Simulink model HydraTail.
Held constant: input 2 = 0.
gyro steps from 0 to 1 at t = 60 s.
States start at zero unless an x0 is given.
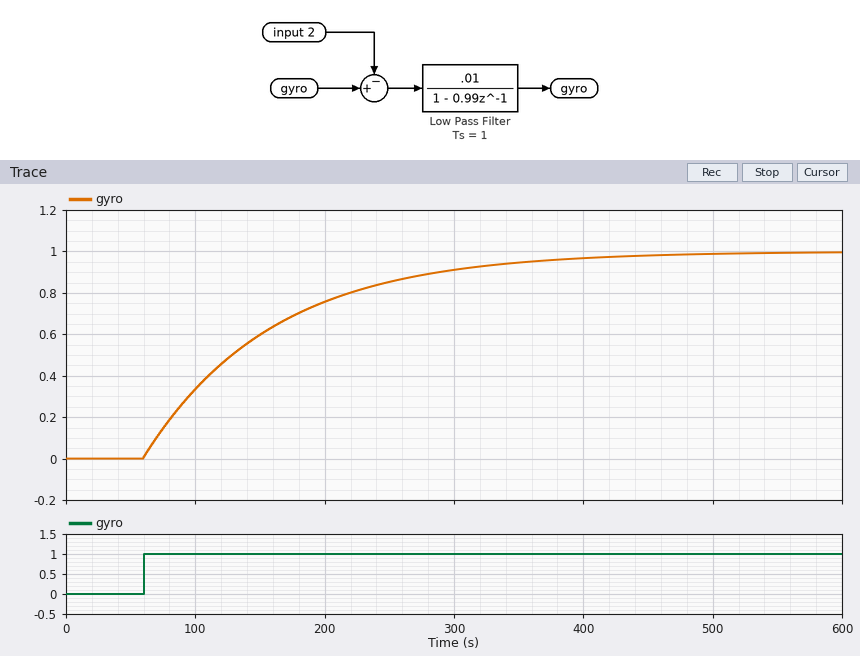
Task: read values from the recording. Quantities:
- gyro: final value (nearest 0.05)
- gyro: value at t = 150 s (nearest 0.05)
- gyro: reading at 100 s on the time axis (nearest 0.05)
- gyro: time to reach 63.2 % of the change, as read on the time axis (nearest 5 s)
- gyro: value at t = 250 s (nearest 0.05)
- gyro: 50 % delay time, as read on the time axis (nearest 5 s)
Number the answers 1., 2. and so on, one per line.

1. 1.00
2. 0.60
3. 0.35
4. 160 s
5. 0.85
6. 130 s
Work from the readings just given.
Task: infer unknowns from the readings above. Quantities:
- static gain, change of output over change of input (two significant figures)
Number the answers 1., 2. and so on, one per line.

1. 1.0
